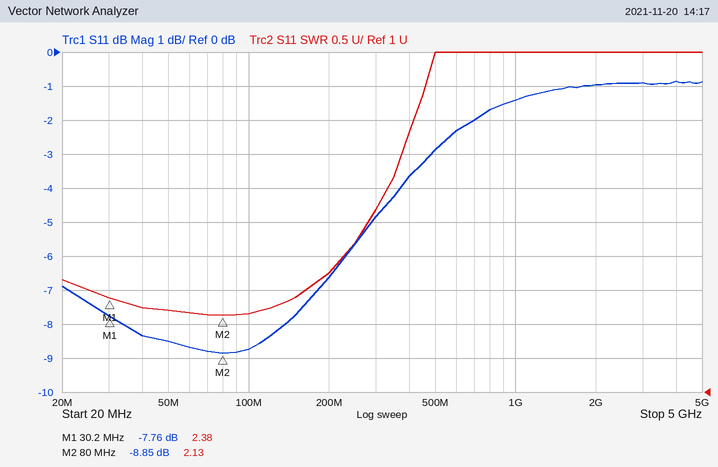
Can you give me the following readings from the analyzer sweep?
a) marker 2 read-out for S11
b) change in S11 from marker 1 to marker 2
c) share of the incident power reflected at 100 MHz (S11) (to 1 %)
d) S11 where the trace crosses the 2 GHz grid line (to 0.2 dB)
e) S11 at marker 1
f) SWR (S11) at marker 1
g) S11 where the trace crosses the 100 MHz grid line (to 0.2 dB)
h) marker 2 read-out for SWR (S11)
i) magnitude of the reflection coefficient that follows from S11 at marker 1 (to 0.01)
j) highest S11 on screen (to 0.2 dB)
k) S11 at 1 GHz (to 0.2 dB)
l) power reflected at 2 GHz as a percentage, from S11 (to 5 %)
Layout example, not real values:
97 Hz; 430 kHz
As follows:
-8.85 dB; -1.09 dB; 13 %; -1.0 dB; -7.76 dB; 2.38; -8.8 dB; 2.13; 0.41; -0.8 dB; -1.4 dB; 80 %
